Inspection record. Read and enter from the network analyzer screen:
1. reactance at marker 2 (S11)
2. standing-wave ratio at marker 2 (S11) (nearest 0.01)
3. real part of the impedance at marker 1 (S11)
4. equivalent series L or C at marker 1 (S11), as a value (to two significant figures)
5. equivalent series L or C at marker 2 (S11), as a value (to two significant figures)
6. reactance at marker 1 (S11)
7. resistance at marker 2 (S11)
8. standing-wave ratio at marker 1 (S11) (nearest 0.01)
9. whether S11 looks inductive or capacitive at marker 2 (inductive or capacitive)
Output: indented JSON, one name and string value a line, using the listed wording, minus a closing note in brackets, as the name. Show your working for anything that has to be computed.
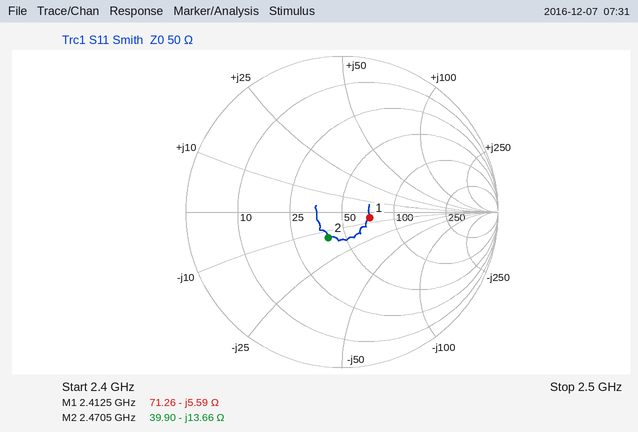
{
  "reactance at marker 2": "-13.66 Ω",
  "standing-wave ratio at marker 2 (S11)": "1.46",
  "real part of the impedance at marker 1": "71.26 Ω",
  "equivalent series L or C at marker 1 (S11), as a value": "C = 1/(2π × 2.4125 GHz × 5.59 Ω) ≈ 12 pF",
  "equivalent series L or C at marker 2 (S11), as a value": "C = 1/(2π × 2.4705 GHz × 13.66 Ω) ≈ 4.7 pF",
  "reactance at marker 1": "-5.59 Ω",
  "resistance at marker 2": "39.90 Ω",
  "standing-wave ratio at marker 1 (S11)": "1.44",
  "whether S11 looks inductive or capacitive at marker 2": "capacitive"
}
